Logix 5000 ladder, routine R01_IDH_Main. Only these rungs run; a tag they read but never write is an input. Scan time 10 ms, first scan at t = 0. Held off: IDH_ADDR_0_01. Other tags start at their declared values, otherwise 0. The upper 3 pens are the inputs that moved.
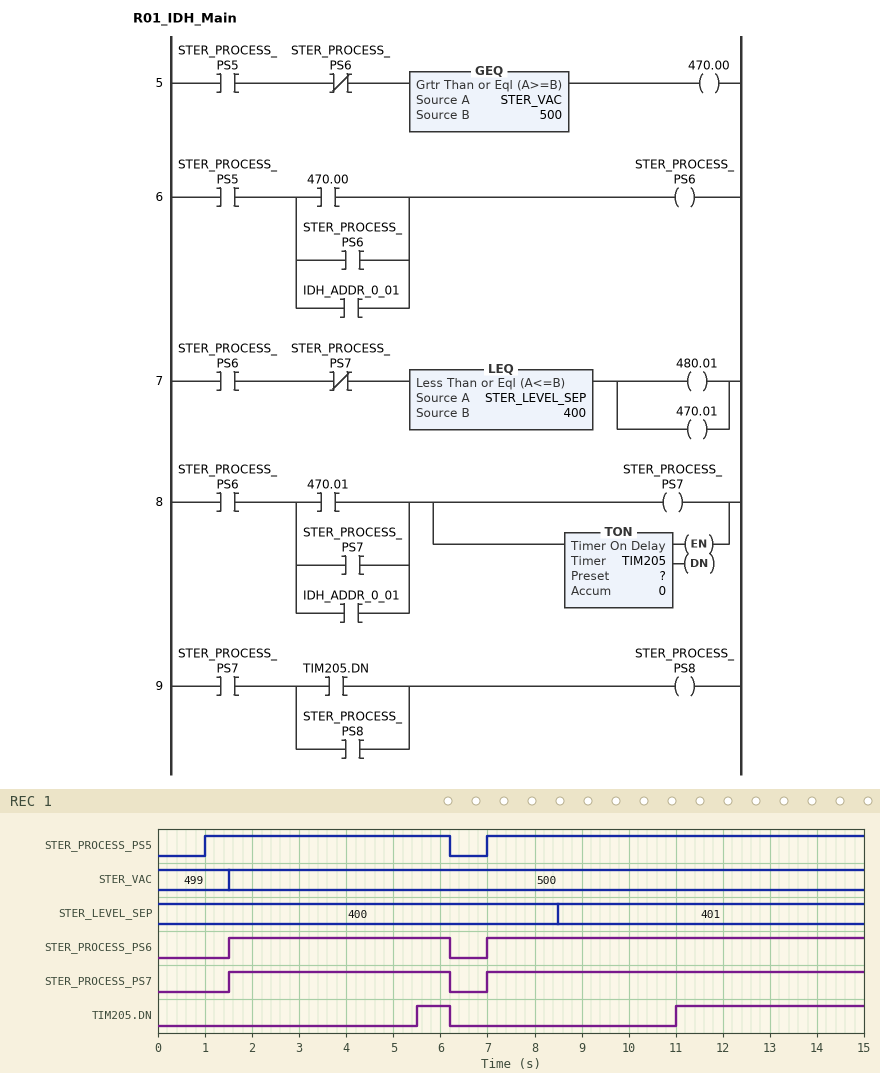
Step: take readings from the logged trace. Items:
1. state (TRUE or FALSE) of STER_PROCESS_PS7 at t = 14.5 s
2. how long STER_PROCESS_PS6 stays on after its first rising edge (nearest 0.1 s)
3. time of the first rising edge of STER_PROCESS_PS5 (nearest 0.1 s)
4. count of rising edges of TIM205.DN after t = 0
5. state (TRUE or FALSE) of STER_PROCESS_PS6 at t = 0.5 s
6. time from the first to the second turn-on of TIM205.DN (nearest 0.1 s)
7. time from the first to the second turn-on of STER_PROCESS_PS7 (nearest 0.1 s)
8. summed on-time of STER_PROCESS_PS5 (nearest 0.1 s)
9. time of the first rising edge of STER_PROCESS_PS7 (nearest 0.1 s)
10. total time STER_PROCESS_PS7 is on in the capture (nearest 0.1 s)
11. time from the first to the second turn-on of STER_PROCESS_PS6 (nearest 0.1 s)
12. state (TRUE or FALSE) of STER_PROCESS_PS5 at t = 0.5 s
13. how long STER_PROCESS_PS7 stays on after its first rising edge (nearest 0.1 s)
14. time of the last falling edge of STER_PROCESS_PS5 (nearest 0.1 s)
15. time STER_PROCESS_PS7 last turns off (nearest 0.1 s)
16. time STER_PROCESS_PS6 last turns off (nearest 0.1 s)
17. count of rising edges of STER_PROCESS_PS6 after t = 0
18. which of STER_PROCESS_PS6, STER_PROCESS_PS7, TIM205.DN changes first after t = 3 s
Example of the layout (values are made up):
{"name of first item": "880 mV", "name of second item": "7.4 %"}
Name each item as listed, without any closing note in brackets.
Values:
{"state (TRUE or FALSE) of STER_PROCESS_PS7 at t = 14.5 s": "TRUE", "how long STER_PROCESS_PS6 stays on after its first rising edge": "4.7 s", "time of the first rising edge of STER_PROCESS_PS5": "1.0 s", "count of rising edges of TIM205.DN after t = 0": "2", "state (TRUE or FALSE) of STER_PROCESS_PS6 at t = 0.5 s": "FALSE", "time from the first to the second turn-on of TIM205.DN": "5.5 s", "time from the first to the second turn-on of STER_PROCESS_PS7": "5.5 s", "summed on-time of STER_PROCESS_PS5": "13.2 s", "time of the first rising edge of STER_PROCESS_PS7": "1.5 s", "total time STER_PROCESS_PS7 is on in the capture": "12.7 s", "time from the first to the second turn-on of STER_PROCESS_PS6": "5.5 s", "state (TRUE or FALSE) of STER_PROCESS_PS5 at t = 0.5 s": "FALSE", "how long STER_PROCESS_PS7 stays on after its first rising edge": "4.7 s", "time of the last falling edge of STER_PROCESS_PS5": "6.2 s", "time STER_PROCESS_PS7 last turns off": "6.2 s", "time STER_PROCESS_PS6 last turns off": "6.2 s", "count of rising edges of STER_PROCESS_PS6 after t = 0": "2", "which of STER_PROCESS_PS6, STER_PROCESS_PS7, TIM205.DN changes first after t = 3 s": "TIM205.DN"}
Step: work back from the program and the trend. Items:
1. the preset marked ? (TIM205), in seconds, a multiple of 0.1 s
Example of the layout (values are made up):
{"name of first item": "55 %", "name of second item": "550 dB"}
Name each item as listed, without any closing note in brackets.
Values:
{"the preset marked ? (TIM205), in seconds, a multiple of 0.1 s": "4.0 s"}
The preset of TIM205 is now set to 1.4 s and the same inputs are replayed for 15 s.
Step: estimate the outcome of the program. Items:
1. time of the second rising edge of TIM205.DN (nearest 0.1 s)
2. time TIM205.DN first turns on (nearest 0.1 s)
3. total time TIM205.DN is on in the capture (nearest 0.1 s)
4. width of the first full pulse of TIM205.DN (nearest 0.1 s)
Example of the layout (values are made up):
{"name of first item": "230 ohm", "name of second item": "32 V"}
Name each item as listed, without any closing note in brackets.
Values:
{"time of the second rising edge of TIM205.DN": "8.4 s", "time TIM205.DN first turns on": "2.9 s", "total time TIM205.DN is on in the capture": "9.9 s", "width of the first full pulse of TIM205.DN": "3.3 s"}
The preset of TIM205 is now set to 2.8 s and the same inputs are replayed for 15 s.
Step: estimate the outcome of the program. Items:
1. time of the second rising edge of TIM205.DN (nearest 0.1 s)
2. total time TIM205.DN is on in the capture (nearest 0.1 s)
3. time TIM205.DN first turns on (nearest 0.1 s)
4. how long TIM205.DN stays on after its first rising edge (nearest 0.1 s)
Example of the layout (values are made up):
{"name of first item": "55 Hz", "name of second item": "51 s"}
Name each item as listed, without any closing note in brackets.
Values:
{"time of the second rising edge of TIM205.DN": "9.8 s", "total time TIM205.DN is on in the capture": "7.1 s", "time TIM205.DN first turns on": "4.3 s", "how long TIM205.DN stays on after its first rising edge": "1.9 s"}
